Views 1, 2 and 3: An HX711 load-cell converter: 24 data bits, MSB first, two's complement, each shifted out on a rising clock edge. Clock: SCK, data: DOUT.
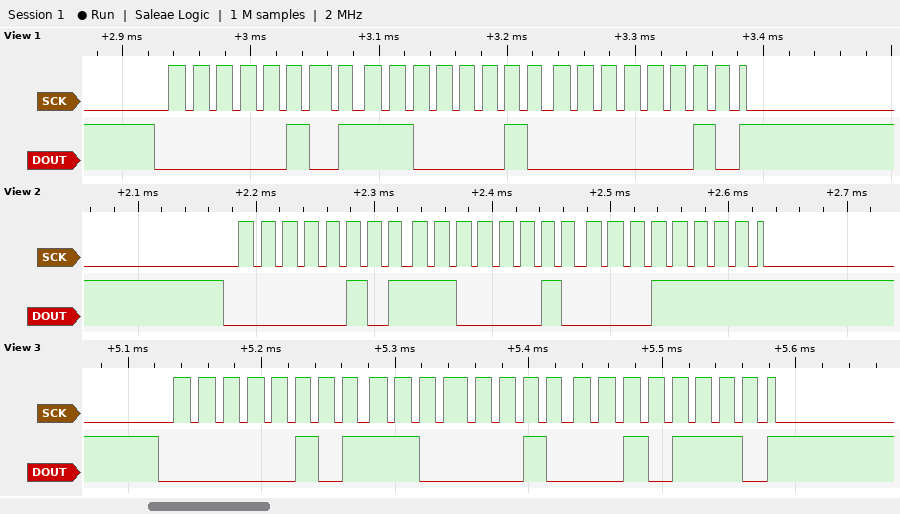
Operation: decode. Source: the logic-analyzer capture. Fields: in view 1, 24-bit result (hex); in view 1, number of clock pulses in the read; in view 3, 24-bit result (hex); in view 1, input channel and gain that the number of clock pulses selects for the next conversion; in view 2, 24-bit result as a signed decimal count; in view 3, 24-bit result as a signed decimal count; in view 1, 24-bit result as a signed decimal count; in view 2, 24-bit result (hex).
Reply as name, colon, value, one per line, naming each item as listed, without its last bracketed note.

in view 1, 24-bit result: 0x05C202
in view 1, number of clock pulses in the read: 25
in view 3, 24-bit result: 0x05C22E
in view 1, input channel and gain that the number of clock pulses selects for the next conversion: channel A, gain 128
in view 2, 24-bit result as a signed decimal count: 377375
in view 3, 24-bit result as a signed decimal count: 377390
in view 1, 24-bit result as a signed decimal count: 377346
in view 2, 24-bit result: 0x05C21F
